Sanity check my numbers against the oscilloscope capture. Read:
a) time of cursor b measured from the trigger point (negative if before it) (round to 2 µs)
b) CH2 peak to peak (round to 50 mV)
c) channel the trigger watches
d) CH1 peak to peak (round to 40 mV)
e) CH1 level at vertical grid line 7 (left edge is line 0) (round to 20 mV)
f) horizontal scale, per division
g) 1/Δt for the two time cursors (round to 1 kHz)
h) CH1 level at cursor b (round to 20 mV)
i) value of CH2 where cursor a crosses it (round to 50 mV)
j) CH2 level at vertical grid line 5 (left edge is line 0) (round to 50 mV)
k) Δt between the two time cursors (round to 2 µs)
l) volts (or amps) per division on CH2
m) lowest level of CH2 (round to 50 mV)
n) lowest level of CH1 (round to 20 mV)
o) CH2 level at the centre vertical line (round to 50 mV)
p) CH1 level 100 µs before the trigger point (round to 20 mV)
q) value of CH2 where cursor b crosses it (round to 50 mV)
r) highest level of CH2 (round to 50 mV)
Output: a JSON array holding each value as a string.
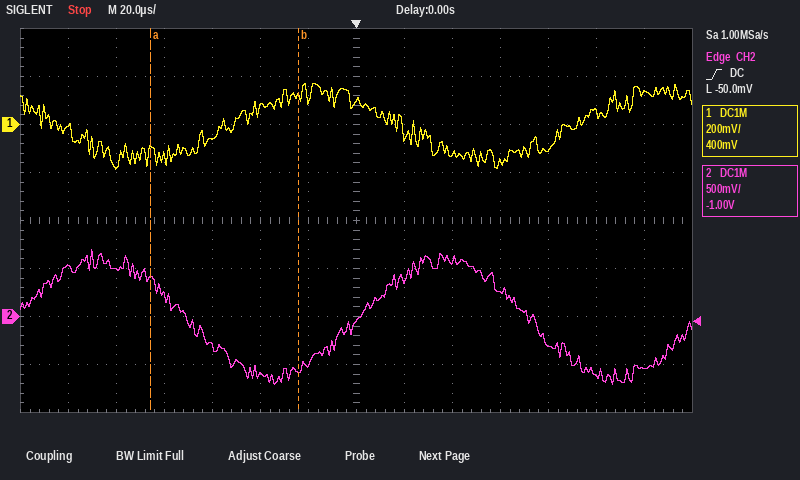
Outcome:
["-24 µs", "1.40 V", "CH2", "360 mV", "100 mV", "20 µs", "16 kHz", "120 mV", "400 mV", "-600 mV", "62 µs", "500 mV", "-700 mV", "-180 mV", "-50 mV", "-180 mV", "-550 mV", "700 mV"]
